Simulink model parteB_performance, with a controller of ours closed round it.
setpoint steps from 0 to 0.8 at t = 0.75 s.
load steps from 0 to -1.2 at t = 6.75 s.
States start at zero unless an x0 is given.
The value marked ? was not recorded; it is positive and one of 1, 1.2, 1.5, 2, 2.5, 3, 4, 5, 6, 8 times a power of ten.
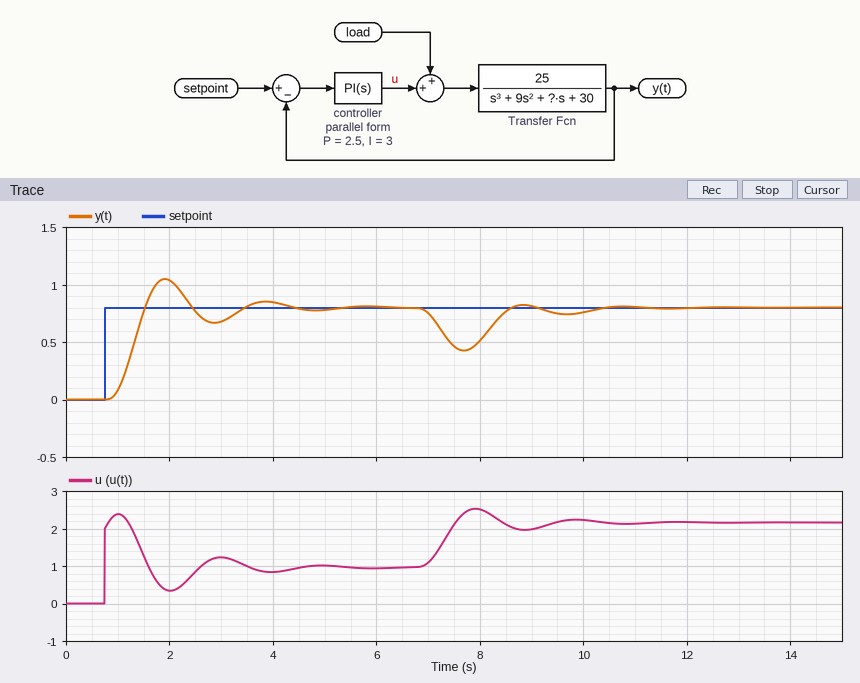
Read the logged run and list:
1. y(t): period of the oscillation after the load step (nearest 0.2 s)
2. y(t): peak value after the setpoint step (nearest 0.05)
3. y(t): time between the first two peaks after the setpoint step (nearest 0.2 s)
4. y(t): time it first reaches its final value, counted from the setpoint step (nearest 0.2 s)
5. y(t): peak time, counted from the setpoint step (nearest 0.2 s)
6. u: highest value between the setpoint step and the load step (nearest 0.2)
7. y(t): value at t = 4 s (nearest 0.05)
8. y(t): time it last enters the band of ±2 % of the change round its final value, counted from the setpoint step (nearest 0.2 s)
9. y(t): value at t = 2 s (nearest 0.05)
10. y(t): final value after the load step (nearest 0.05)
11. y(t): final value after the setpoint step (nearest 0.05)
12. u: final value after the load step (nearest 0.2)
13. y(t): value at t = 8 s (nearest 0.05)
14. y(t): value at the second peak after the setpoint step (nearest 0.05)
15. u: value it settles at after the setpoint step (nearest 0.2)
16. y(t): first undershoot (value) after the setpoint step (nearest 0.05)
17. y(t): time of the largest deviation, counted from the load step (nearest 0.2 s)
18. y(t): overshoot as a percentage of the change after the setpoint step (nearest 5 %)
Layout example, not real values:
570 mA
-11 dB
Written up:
2.0 s
1.05
2.0 s
0.8 s
1.2 s
2.4
0.85
4.4 s
1.05
0.80
0.80
2.2
0.50
0.85
1.0
0.65
1.0 s
30 %
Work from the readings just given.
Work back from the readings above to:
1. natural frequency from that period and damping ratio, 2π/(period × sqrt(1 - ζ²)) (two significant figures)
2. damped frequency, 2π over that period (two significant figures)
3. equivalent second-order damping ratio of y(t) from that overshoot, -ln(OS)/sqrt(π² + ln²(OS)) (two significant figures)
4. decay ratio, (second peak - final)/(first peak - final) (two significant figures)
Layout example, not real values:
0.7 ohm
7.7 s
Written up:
3.4 rad/s
3.1 rad/s
0.36
0.20
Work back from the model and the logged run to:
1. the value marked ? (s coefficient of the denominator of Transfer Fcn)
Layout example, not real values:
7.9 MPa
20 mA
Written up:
30
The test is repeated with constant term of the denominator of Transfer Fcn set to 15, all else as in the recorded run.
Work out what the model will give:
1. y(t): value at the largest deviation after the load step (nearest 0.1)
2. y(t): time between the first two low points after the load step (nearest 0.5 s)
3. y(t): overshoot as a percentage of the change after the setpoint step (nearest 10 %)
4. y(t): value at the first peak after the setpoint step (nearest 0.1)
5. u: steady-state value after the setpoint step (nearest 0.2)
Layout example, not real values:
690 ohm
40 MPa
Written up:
0.4
2.5 s
50 %
1.2
0.4
